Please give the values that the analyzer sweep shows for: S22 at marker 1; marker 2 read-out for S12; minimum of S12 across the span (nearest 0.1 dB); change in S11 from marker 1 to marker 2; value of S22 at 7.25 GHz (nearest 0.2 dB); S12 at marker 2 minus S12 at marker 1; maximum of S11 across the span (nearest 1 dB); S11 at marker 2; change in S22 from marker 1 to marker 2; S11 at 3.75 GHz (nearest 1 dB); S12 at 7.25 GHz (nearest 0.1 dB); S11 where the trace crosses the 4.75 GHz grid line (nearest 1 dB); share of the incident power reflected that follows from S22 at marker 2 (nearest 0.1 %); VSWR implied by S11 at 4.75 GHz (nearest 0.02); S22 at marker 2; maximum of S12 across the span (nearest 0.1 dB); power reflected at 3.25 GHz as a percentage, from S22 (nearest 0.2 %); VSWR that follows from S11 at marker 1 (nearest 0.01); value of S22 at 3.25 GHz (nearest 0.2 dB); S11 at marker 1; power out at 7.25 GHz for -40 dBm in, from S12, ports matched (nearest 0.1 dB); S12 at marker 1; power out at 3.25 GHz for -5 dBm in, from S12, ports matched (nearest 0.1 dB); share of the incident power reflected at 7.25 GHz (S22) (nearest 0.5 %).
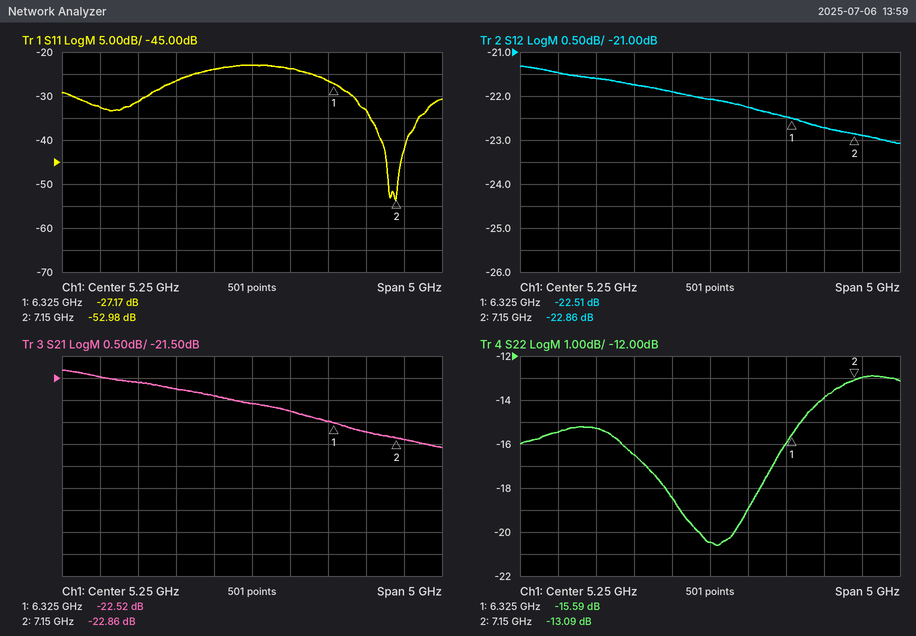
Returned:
-15.59 dB
-22.86 dB
-23.1 dB
-25.81 dB
-13.0 dB
-0.35 dB
-23 dB
-52.98 dB
2.50 dB
-31 dB
-22.9 dB
-24 dB
4.9 %
1.14
-13.09 dB
-21.3 dB
2.8 %
1.09
-15.4 dB
-27.17 dB
-62.9 dBm
-22.51 dB
-26.5 dBm
5.0 %
